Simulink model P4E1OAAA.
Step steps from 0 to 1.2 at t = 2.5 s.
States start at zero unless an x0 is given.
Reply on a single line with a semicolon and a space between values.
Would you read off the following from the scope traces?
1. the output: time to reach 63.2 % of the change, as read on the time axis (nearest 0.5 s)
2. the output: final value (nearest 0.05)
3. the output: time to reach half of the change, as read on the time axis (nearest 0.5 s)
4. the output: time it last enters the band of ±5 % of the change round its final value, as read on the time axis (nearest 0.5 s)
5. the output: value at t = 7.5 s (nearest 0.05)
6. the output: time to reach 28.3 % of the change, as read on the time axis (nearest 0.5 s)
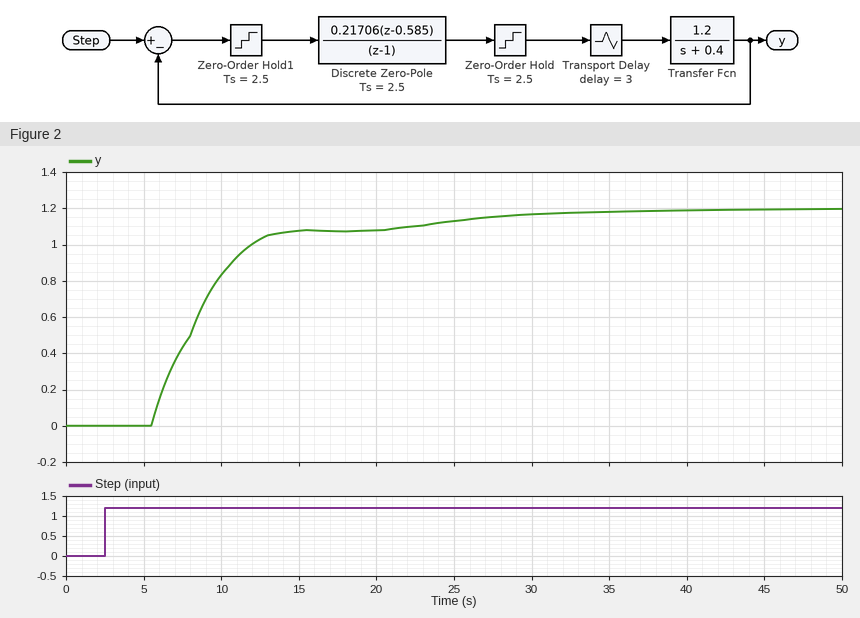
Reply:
9.5 s; 1.20; 8.5 s; 26.0 s; 0.45; 7.0 s
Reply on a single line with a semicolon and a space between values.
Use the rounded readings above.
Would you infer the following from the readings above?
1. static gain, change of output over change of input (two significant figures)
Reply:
1.0
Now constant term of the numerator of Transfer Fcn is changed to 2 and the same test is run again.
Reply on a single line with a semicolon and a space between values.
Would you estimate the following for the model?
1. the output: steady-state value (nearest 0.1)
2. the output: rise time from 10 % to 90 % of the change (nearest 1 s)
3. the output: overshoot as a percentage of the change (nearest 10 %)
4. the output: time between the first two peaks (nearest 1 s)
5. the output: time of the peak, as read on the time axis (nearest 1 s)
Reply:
1.2; 3 s; 30 %; 15 s; 13 s
